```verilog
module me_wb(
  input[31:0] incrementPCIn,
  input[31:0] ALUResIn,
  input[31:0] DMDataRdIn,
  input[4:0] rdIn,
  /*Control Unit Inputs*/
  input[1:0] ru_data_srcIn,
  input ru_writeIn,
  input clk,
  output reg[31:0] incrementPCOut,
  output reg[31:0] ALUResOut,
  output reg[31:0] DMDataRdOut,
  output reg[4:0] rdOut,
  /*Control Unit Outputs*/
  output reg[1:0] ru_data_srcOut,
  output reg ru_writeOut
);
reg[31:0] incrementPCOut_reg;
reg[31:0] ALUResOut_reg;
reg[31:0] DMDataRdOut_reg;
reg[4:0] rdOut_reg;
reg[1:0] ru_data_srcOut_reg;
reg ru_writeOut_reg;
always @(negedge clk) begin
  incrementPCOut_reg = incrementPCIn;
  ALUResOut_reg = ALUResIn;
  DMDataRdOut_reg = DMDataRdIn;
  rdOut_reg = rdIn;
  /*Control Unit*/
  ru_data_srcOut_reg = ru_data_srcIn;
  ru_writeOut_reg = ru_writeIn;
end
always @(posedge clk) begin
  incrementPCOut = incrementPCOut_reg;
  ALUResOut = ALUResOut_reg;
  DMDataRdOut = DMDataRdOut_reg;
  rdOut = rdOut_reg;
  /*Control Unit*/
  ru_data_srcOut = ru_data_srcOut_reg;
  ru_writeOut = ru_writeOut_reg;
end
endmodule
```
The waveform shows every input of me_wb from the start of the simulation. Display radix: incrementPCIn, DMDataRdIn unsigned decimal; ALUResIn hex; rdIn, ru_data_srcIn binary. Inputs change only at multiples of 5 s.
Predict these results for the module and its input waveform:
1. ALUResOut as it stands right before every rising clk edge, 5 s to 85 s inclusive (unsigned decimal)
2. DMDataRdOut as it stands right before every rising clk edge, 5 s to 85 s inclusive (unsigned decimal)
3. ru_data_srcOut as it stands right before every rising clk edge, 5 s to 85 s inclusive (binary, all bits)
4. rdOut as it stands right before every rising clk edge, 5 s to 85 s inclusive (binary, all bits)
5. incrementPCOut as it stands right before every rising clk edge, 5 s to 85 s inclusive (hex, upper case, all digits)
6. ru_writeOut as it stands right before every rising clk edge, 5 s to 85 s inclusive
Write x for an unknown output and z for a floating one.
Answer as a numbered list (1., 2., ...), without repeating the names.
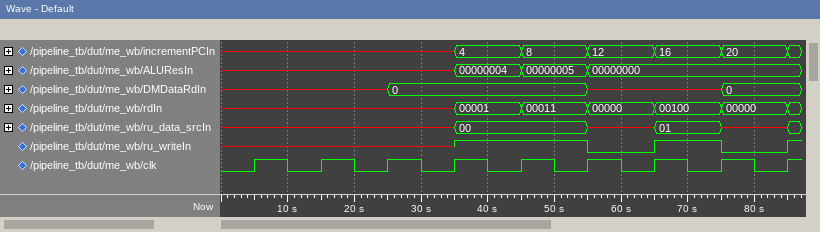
1. x, x, x, x, x, 4, 5, 0, 0
2. x, x, x, x, 0, 0, 0, x, x
3. x, x, x, x, x, 00, 00, x, 01
4. x, x, x, x, x, 00001, 00011, 00000, 00100
5. x, x, x, x, x, 00000004, 00000008, 0000000C, 00000010
6. x x x x x 1 1 0 1
